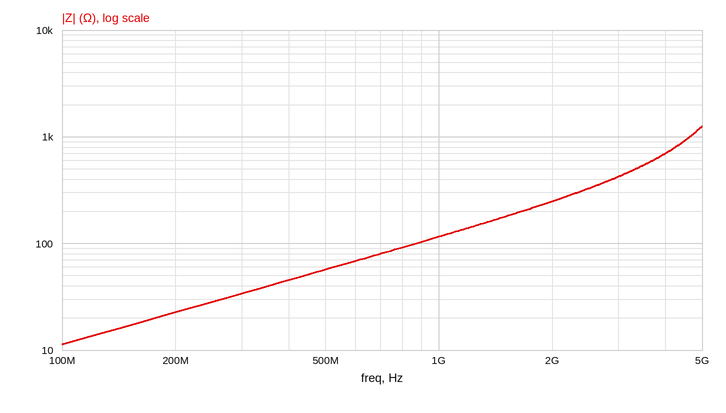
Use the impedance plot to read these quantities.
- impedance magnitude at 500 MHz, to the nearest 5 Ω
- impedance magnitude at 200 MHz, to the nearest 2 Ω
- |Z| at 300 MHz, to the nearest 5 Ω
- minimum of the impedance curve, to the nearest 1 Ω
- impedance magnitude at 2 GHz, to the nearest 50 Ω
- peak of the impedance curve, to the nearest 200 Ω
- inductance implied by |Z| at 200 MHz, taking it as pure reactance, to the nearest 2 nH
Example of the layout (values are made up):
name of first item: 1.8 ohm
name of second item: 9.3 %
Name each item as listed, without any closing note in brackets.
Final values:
impedance magnitude at 500 MHz, to the nearest 5 Ω: 55 Ω
impedance magnitude at 200 MHz, to the nearest 2 Ω: 22 Ω
|Z| at 300 MHz, to the nearest 5 Ω: 35 Ω
minimum of the impedance curve, to the nearest 1 Ω: 11 Ω
impedance magnitude at 2 GHz, to the nearest 50 Ω: 250 Ω
peak of the impedance curve, to the nearest 200 Ω: 1.2 kΩ
inductance implied by |Z| at 200 MHz, taking it as pure reactance, to the nearest 2 nH: 18 nH
